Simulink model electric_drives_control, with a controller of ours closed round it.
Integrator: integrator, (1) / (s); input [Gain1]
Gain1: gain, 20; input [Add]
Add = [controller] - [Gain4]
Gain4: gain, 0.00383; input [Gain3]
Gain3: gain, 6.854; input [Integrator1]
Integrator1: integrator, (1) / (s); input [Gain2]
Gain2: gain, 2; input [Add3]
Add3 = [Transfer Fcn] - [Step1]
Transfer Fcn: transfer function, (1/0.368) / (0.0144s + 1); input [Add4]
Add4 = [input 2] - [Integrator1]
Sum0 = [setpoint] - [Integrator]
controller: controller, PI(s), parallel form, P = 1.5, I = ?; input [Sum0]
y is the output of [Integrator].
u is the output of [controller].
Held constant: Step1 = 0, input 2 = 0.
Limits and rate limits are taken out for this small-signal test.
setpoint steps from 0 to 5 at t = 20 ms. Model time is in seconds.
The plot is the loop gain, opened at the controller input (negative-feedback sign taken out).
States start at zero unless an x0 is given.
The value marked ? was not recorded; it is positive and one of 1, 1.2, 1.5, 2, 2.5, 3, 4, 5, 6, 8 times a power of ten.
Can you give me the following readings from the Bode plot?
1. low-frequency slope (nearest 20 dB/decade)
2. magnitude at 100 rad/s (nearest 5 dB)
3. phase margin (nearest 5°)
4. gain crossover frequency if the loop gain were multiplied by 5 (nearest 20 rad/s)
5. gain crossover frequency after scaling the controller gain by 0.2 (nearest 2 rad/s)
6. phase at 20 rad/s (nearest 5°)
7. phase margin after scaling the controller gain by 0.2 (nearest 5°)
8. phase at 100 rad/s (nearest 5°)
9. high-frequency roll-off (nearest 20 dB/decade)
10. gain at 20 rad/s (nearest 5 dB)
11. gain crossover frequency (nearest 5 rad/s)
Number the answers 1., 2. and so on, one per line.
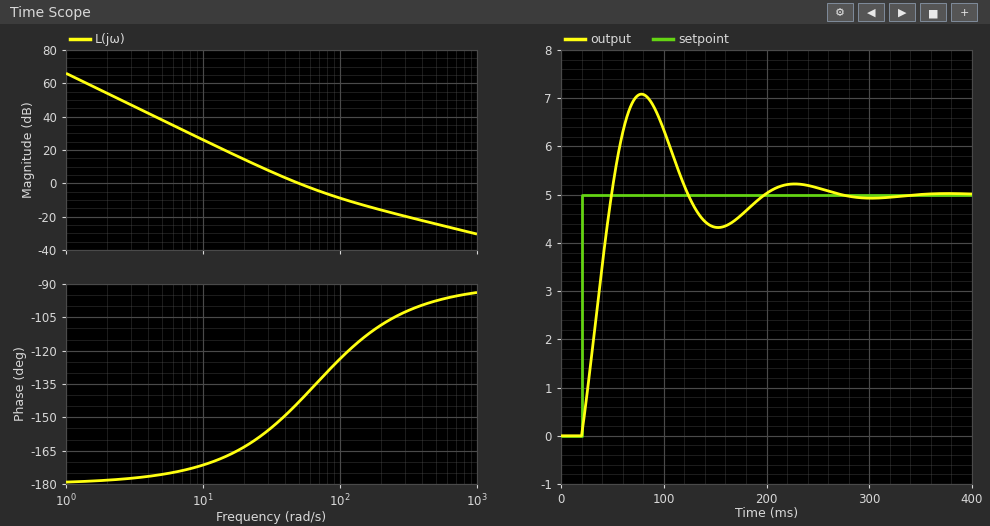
1. -40 dB/decade
2. -10 dB
3. 35°
4. 160 rad/s
5. 20 rad/s
6. -165°
7. 15°
8. -125°
9. -20 dB/decade
10. 15 dB
11. 50 rad/s
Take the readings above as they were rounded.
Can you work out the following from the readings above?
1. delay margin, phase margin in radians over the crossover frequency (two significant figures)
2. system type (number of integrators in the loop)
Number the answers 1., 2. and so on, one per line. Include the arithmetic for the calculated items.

1. 35 × π / 180 / 50 = 0.012 s
2. 2
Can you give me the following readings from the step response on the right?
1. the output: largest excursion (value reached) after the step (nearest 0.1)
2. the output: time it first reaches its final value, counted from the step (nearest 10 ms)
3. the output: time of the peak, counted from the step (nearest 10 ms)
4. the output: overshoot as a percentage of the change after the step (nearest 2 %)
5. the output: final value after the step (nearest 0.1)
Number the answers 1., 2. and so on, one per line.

1. 7.1
2. 30 ms
3. 60 ms
4. 42 %
5. 5.0
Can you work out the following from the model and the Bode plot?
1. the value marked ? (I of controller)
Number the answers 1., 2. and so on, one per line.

1. 100
